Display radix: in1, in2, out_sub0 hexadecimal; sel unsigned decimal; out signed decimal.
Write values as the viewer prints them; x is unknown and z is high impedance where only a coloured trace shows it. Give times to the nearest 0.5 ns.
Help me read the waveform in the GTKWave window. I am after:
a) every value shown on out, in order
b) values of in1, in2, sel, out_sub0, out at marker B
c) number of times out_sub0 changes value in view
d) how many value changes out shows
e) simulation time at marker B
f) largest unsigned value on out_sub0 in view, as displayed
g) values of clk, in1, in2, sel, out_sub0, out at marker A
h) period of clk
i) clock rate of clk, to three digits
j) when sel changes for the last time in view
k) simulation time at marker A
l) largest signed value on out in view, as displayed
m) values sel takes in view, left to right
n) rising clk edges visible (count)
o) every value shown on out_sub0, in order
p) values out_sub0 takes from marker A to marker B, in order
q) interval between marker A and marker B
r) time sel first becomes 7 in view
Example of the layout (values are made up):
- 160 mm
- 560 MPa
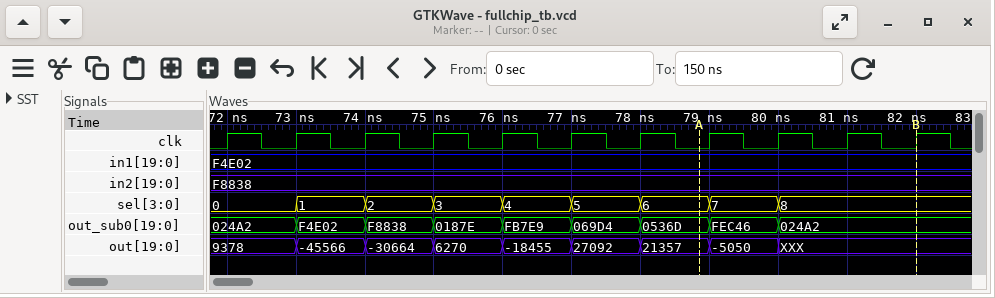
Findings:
- 9378, -45566, -30664, 6270, -18455, 27092, 21357, -5050, XXX
- in1=F4E02, in2=F8838, sel=8, out_sub0=024A2, out=XXX
- 8
- 8
- 82 ns
- FEC46
- clk=0, in1=F4E02, in2=F8838, sel=6, out_sub0=0536D, out=21357
- 1 ns
- 1.00 GHz
- 80 ns
- 79 ns
- 27092
- 0, 1, 2, 3, 4, 5, 6, 7, 8
- 11
- 024A2, F4E02, F8838, 0187E, FB7E9, 069D4, 0536D, FEC46, 024A2
- 0536D, FEC46, 024A2
- 3 ns
- 79 ns
